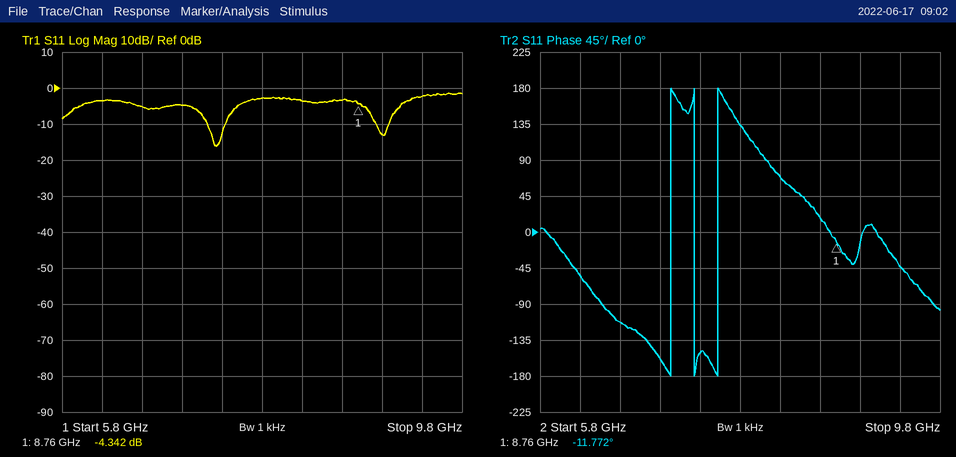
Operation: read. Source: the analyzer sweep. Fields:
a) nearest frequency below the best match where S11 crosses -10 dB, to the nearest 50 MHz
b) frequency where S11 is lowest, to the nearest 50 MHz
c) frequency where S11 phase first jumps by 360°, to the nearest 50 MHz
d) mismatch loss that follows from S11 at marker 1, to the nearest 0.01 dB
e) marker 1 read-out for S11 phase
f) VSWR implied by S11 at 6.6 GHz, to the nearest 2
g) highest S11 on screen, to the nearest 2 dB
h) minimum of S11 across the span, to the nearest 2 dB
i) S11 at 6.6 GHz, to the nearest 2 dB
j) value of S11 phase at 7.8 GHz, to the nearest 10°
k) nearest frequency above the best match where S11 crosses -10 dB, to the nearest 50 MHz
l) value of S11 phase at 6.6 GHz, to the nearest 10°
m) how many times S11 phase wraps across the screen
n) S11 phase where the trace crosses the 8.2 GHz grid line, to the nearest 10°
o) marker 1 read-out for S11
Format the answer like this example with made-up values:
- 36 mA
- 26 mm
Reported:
- 7.25 GHz
- 7.35 GHz
- 7.10 GHz
- 1.99 dB
- -11.772°
- 4
- -2 dB
- -16 dB
- -6 dB
- 130°
- 7.45 GHz
- -110°
- 3
- 70°
- -4.342 dB
